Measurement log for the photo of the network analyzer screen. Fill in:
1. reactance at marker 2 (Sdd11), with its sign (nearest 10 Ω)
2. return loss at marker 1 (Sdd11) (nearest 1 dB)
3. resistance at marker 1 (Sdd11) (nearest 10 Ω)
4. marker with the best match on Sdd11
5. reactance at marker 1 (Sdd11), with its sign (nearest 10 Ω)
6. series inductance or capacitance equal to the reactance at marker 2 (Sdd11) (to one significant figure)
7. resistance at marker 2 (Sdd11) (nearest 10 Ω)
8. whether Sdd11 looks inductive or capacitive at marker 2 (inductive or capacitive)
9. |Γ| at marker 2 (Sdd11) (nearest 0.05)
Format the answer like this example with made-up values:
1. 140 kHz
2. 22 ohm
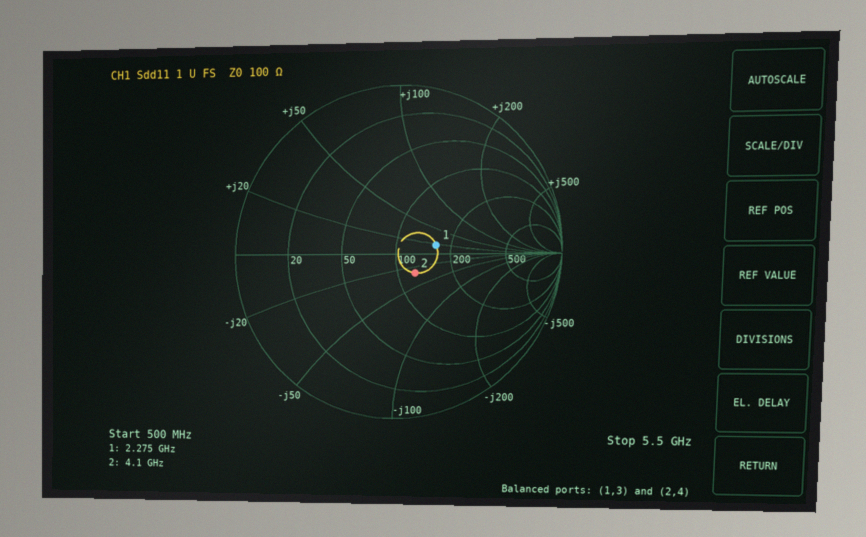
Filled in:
1. -30 Ω
2. 12 dB
3. 160 Ω
4. marker 2
5. +20 Ω
6. 1 pF
7. 120 Ω
8. capacitive
9. 0.15
